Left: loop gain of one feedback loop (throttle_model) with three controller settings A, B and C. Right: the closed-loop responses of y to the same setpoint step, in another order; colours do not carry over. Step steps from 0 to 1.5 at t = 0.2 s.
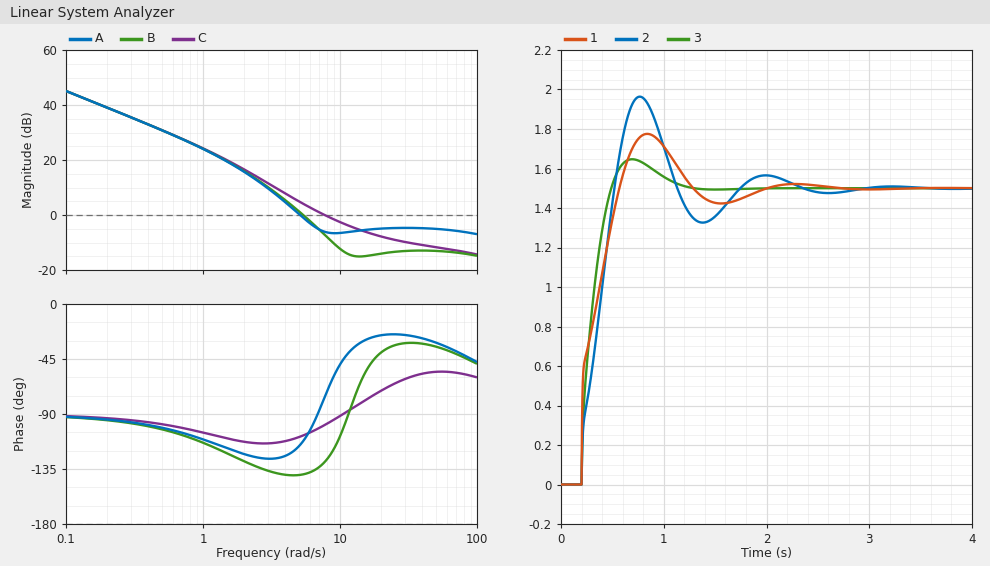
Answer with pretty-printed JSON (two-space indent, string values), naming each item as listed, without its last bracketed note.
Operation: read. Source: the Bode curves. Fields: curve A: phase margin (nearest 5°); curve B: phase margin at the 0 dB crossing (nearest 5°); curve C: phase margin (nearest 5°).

{
  "curve A: phase margin": "65°",
  "curve B: phase margin at the 0 dB crossing": "40°",
  "curve C: phase margin": "80°"
}
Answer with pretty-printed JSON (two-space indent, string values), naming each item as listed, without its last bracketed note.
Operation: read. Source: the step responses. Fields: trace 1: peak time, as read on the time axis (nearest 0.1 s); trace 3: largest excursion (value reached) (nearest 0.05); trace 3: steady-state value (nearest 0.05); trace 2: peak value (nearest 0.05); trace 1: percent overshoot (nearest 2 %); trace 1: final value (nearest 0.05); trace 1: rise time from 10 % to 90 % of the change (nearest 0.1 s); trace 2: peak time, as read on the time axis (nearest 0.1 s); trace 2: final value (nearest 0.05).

{
  "trace 1: peak time, as read on the time axis": "0.8 s",
  "trace 3: largest excursion (value reached)": "1.65",
  "trace 3: steady-state value": "1.50",
  "trace 2: peak value": "1.95",
  "trace 1: percent overshoot": "18 %",
  "trace 1: final value": "1.50",
  "trace 1: rise time from 10 % to 90 % of the change": "0.3 s",
  "trace 2: peak time, as read on the time axis": "0.8 s",
  "trace 2: final value": "1.50"
}
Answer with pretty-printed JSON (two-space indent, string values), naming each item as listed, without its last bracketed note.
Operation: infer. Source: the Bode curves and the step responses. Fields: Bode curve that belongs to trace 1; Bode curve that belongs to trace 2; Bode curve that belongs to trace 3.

{
  "Bode curve that belongs to trace 1": "A",
  "Bode curve that belongs to trace 2": "B",
  "Bode curve that belongs to trace 3": "C"
}
